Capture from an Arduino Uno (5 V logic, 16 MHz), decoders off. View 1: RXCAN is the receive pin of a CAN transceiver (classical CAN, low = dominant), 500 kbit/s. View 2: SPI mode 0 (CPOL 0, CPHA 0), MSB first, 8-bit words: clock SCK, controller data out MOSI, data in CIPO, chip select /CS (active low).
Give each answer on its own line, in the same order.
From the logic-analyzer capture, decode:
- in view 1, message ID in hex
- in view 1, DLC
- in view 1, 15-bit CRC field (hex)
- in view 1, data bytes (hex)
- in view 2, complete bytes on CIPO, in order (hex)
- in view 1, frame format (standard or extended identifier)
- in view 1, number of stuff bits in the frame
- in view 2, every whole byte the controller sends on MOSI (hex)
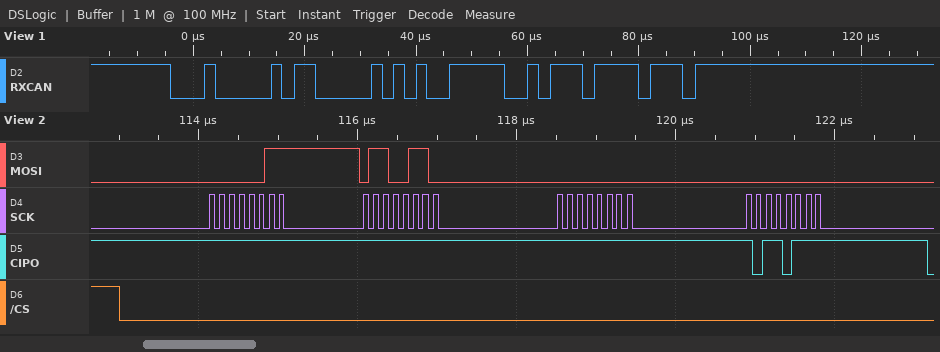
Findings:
0x103
1
0x577B
4F
FF FF FF B7
standard
3
03 66 00 00
